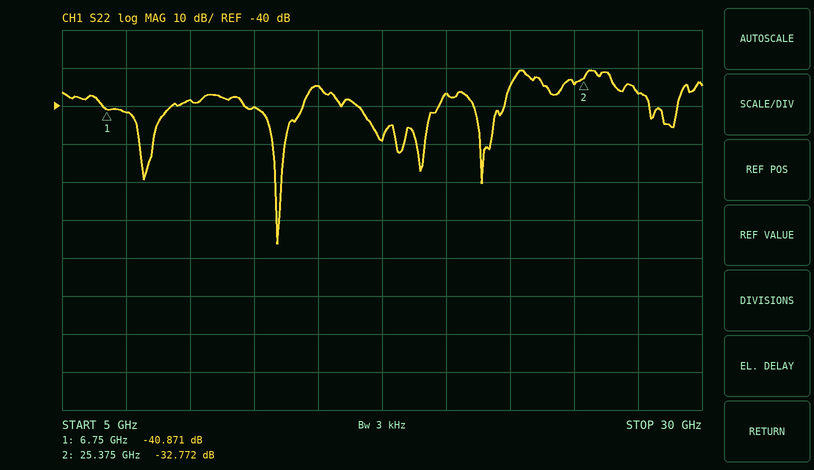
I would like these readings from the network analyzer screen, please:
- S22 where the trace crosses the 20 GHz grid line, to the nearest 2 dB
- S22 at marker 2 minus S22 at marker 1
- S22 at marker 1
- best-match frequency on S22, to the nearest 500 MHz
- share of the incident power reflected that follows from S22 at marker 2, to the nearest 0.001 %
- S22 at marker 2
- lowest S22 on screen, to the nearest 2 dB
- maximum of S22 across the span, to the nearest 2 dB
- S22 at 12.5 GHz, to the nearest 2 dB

-36 dB
8.099 dB
-40.871 dB
13.5 GHz
0.053 %
-32.772 dB
-76 dB
-30 dB
-40 dB
